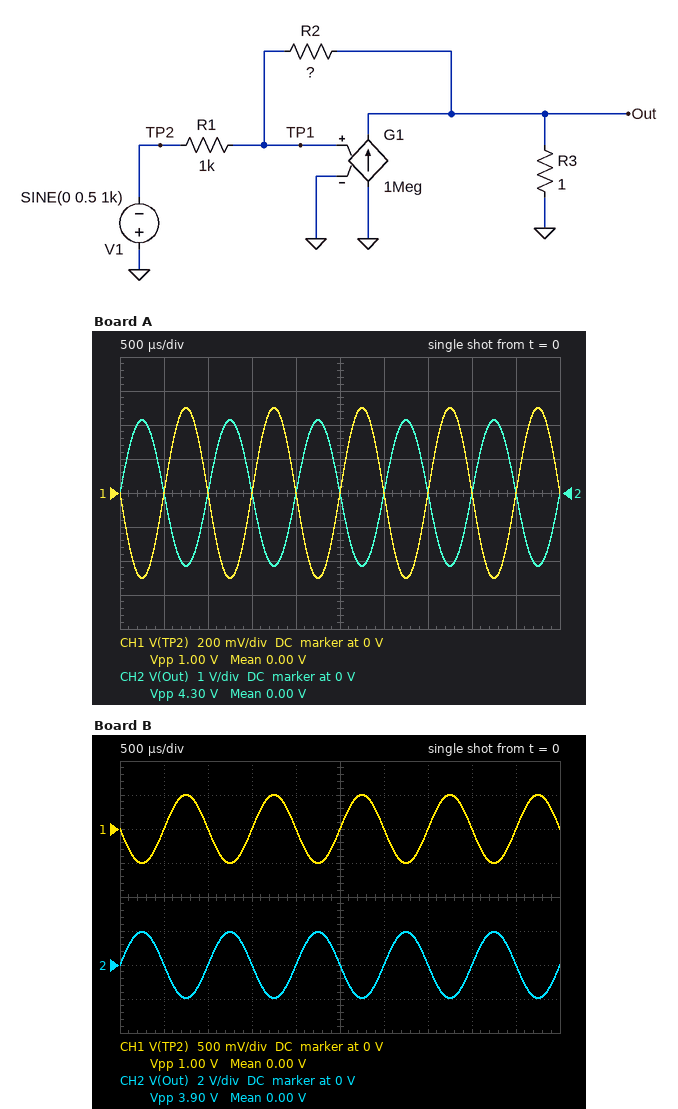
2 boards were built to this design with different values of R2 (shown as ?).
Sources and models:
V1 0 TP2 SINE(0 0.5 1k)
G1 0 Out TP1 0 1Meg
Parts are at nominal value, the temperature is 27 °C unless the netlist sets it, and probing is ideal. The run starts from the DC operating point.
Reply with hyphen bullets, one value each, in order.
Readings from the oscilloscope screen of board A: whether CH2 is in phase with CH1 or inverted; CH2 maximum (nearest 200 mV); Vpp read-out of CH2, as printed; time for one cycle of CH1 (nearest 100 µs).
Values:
- inverted
- 2.2 V
- 4.30 V
- 1.0 ms
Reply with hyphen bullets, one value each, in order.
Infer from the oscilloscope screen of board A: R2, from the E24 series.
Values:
- 4.3 kΩ
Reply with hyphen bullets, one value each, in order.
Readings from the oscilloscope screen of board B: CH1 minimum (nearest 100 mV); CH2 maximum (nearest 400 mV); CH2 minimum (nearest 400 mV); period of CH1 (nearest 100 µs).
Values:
- -500 mV
- 2.0 V
- -2.0 V
- 1.0 ms
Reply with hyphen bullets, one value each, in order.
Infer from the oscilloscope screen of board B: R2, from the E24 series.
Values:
- 3.9 kΩ
